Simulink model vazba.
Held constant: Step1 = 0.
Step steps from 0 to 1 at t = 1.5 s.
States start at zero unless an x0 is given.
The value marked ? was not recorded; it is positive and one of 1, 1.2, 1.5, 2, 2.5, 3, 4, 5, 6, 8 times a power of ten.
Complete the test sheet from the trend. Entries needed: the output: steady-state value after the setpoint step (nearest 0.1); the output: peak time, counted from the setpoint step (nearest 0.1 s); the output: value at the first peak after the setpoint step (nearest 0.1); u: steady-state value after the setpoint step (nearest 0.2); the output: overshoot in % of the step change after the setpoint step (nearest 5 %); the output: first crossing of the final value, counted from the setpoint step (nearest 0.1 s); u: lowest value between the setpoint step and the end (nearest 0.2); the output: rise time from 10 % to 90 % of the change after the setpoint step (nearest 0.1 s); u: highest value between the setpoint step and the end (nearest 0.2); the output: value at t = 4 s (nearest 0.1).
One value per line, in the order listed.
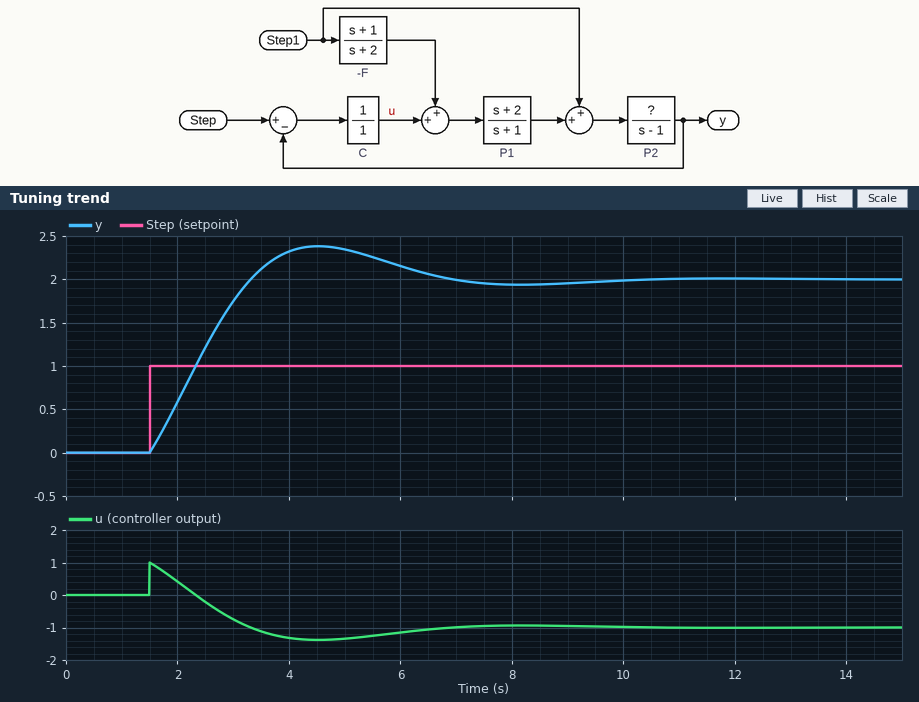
2.0
3.0 s
2.4
-1.0
20 %
1.8 s
-1.4
1.4 s
1.0
2.3
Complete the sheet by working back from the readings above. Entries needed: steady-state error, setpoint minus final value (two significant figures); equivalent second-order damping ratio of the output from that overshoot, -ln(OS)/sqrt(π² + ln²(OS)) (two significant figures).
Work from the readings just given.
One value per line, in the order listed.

-1.0
0.46
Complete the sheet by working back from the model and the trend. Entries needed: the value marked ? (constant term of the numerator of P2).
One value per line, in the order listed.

1
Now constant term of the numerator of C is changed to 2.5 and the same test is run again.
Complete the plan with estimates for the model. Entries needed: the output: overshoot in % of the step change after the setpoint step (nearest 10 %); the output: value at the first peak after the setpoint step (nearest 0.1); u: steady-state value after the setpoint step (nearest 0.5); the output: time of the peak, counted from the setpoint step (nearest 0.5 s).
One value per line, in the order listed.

20 %
1.5
-0.5
1.5 s
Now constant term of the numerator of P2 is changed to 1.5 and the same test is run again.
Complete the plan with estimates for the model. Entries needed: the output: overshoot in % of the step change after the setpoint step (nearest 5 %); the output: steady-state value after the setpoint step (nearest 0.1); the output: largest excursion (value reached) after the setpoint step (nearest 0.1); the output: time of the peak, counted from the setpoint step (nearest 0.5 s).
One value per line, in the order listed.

20 %
1.5
1.8
2.0 s
